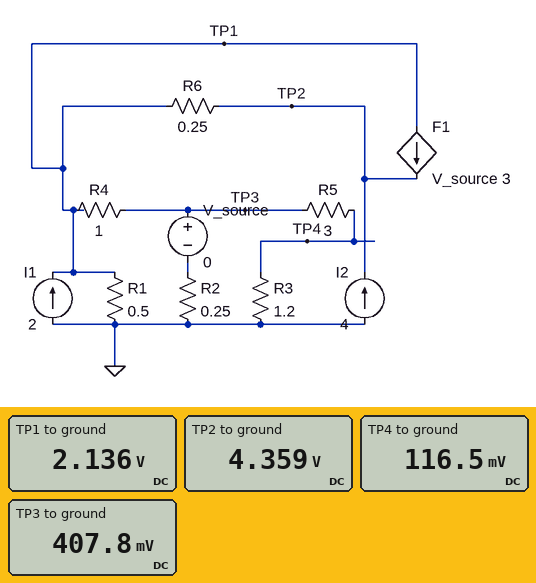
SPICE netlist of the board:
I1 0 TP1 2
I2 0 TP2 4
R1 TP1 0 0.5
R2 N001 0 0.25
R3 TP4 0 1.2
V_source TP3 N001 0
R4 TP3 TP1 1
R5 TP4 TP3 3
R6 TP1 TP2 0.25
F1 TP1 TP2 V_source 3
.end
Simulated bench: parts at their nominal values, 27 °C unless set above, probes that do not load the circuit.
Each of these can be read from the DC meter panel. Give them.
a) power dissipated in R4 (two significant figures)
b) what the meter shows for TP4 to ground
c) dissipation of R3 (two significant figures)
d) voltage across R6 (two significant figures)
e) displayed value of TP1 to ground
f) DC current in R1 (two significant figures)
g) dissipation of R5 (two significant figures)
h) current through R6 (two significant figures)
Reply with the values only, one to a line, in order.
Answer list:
3.0 W
116.5 mV
11 mW
2.2 V
2.136 V
4.3 A
28 mW
8.9 A
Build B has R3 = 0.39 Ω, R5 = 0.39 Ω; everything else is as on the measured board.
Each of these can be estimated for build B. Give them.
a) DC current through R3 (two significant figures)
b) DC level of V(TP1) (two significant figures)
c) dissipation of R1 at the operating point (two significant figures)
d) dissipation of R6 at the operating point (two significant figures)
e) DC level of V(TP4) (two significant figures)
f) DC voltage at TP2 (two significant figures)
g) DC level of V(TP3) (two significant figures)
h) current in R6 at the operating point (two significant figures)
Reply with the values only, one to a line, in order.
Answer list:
430 mA
2.1 V
8.9 W
16 W
170 mV
4.1 V
340 mV
8.0 A
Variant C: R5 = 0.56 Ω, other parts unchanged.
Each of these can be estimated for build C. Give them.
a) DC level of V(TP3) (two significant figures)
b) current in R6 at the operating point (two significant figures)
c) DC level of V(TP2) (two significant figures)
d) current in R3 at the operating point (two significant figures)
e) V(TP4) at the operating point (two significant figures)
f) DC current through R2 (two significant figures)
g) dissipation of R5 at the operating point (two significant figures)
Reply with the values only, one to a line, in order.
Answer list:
380 mV
8.6 A
4.3 V
220 mA
260 mV
1.5 A
26 mW
